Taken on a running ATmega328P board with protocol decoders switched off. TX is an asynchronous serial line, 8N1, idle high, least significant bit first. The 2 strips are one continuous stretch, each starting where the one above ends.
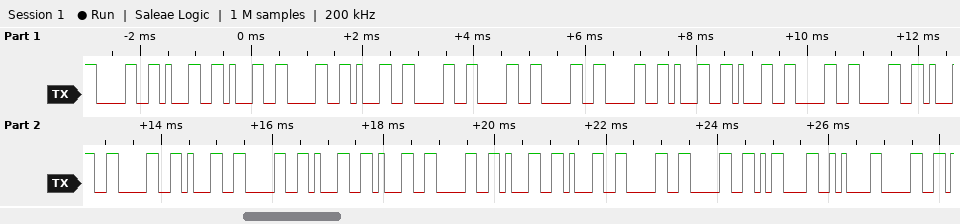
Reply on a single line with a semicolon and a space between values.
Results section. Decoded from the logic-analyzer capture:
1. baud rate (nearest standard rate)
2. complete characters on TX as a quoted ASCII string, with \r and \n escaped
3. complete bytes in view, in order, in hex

9600 baud; "011010000110010101101100\r\n0"; 30 31 31 30 31 30 30 30 30 31 31 30 30 31 30 31 30 31 31 30 31 31 30 30 0D 0A 30
